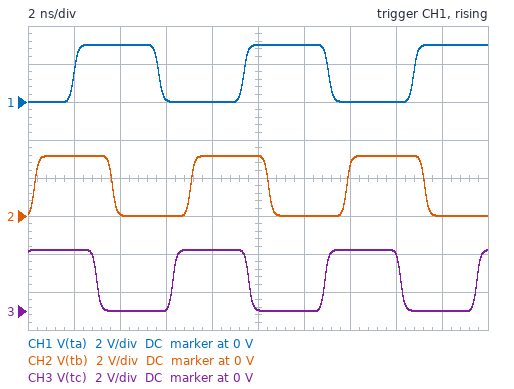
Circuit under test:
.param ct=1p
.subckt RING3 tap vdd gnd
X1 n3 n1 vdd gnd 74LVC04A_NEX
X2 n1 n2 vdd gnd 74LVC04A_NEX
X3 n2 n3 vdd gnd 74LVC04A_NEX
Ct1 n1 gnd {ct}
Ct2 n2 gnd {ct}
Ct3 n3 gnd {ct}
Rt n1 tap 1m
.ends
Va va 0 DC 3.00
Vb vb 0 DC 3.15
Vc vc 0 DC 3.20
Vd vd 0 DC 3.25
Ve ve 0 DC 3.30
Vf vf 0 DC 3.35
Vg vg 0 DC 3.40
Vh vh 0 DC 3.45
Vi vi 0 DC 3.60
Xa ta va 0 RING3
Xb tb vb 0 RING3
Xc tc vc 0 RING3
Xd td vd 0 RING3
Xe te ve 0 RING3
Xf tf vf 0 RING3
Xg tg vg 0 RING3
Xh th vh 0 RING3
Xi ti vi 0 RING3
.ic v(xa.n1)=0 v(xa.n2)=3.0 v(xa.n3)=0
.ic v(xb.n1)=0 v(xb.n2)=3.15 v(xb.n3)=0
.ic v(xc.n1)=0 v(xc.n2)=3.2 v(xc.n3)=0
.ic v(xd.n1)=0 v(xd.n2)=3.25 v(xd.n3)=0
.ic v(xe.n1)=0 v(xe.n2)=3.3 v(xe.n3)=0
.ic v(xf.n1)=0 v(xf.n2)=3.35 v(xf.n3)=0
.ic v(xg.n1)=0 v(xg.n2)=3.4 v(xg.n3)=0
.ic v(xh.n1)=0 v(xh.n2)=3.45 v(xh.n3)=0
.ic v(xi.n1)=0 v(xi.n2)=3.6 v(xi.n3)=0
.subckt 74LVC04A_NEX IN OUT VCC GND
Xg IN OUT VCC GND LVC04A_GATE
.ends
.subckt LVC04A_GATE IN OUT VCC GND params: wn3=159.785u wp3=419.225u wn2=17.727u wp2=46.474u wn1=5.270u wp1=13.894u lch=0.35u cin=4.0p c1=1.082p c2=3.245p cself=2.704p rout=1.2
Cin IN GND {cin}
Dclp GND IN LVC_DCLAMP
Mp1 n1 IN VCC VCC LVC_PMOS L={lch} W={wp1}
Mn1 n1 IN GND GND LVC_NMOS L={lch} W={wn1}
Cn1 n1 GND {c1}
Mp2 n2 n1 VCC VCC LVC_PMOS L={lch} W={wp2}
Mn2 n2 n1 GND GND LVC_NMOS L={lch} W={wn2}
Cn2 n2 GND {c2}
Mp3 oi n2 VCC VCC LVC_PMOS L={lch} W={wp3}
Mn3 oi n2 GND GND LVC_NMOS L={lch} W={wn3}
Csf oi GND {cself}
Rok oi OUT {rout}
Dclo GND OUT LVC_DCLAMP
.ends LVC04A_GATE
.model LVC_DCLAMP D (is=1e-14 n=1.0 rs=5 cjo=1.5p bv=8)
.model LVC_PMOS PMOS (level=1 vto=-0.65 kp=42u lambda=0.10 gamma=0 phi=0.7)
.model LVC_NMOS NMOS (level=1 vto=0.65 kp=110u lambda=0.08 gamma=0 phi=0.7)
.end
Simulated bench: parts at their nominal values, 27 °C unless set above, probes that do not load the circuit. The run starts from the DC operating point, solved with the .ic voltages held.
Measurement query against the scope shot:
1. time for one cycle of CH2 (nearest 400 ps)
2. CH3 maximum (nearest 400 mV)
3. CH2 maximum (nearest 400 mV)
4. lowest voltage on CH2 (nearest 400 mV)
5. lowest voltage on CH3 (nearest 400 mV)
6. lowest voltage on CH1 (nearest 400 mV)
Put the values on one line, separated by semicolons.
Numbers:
6.8 ns; 3.2 V; 3.2 V; 0 V; 0 V; 0 V
